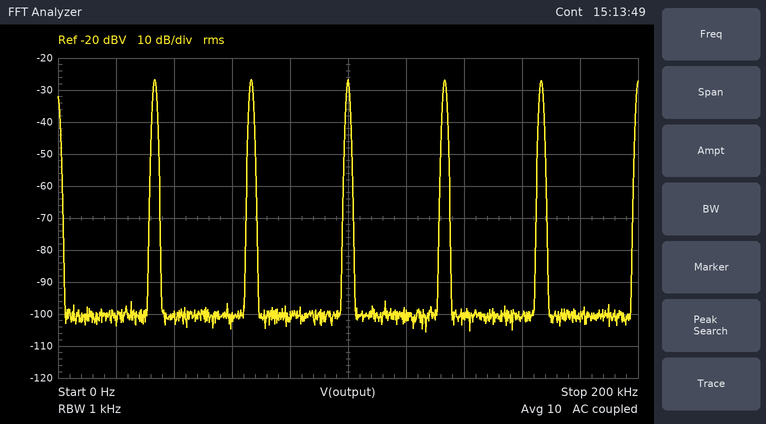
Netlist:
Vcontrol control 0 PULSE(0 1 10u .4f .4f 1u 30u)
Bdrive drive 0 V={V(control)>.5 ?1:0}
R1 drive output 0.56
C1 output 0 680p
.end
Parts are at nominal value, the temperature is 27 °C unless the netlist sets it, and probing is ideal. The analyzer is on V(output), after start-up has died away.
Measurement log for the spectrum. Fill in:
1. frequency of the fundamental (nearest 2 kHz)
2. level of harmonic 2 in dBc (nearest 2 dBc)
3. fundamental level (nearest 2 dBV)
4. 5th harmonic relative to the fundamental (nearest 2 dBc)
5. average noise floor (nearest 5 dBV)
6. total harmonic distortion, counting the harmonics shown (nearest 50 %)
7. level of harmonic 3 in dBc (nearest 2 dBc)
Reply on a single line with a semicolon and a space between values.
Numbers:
34 kHz; 0 dBc; -26 dBV; 0 dBc; -100 dBV; 200 %; 0 dBc
